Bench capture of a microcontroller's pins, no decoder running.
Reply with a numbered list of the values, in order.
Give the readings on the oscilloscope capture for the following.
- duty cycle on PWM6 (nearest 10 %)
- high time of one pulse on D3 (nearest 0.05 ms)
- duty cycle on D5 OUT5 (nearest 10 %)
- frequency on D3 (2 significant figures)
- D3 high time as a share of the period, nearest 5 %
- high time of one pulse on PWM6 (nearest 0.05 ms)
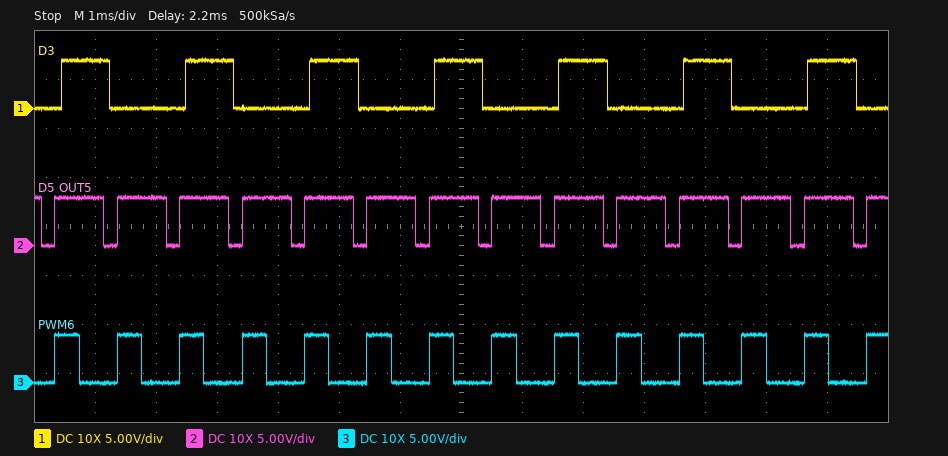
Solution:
1. 40 %
2. 0.80 ms
3. 80 %
4. 490 Hz
5. 40 %
6. 0.40 ms
